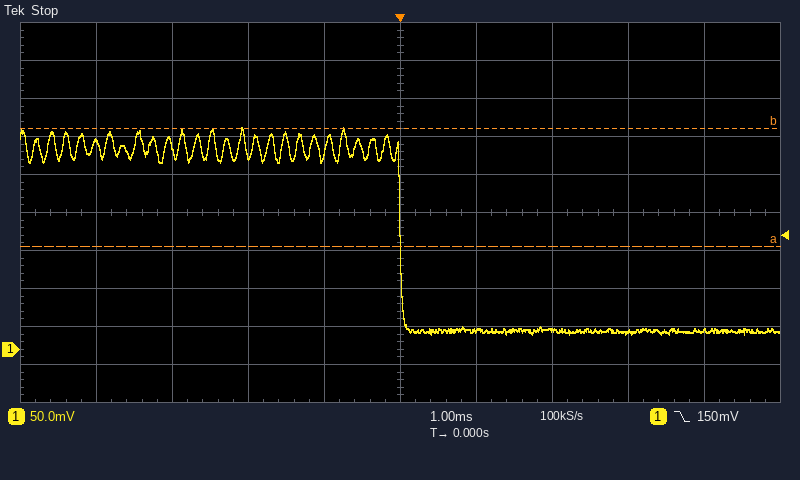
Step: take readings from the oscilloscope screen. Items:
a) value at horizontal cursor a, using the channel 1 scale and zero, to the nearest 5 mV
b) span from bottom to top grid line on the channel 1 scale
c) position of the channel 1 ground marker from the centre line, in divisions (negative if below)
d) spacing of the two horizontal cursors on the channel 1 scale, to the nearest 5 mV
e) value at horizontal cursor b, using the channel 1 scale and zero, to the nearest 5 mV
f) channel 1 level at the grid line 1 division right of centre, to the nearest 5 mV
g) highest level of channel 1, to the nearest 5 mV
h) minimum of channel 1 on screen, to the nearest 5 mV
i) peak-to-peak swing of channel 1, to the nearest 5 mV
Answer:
135 mV
500 mV
-3.6 div
155 mV
290 mV
25 mV
290 mV
20 mV
270 mV
